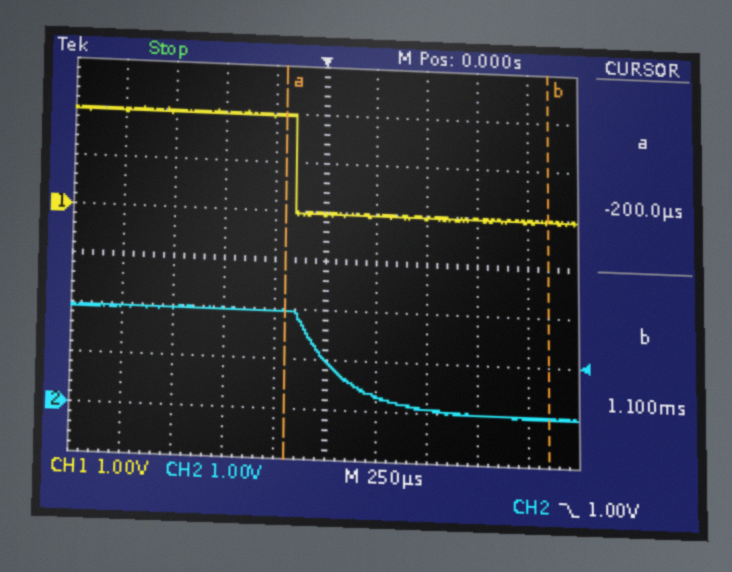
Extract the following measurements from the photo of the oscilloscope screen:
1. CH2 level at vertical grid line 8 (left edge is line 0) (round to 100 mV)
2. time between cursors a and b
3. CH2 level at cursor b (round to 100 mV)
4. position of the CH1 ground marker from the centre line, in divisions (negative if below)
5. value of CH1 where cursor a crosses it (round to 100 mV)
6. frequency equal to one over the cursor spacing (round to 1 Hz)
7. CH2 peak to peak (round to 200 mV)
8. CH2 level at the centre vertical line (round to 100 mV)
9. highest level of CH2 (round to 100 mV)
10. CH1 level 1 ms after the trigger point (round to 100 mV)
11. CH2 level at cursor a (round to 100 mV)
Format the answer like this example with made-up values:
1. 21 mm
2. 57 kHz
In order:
1. 0.0 V
2. 1.300 ms
3. 0.0 V
4. +1.0 div
5. 2.0 V
6. 769 Hz
7. 2.0 V
8. 1.0 V
9. 2.0 V
10. 0.0 V
11. 2.0 V
